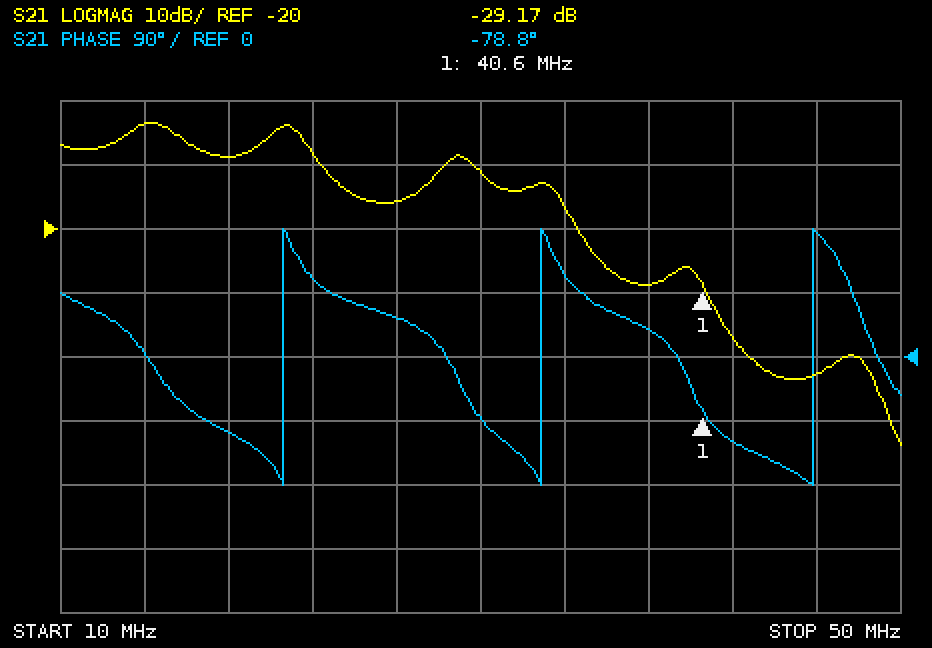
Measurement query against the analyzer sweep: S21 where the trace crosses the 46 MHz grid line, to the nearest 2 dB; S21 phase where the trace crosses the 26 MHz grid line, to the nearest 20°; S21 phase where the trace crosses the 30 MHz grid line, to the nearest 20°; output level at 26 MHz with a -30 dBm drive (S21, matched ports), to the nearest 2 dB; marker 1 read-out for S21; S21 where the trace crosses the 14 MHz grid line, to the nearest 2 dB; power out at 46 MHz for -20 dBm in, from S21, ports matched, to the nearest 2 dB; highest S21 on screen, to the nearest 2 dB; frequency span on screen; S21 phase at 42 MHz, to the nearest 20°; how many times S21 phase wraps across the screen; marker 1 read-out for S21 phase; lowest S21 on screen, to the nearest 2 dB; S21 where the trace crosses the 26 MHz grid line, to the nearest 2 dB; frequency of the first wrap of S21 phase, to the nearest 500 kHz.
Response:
-42 dB
60°
-80°
-46 dBm
-29.17 dB
-4 dB
-62 dBm
-4 dB
40 MHz
-120°
3
-78.8°
-54 dB
-16 dB
20.5 MHz
